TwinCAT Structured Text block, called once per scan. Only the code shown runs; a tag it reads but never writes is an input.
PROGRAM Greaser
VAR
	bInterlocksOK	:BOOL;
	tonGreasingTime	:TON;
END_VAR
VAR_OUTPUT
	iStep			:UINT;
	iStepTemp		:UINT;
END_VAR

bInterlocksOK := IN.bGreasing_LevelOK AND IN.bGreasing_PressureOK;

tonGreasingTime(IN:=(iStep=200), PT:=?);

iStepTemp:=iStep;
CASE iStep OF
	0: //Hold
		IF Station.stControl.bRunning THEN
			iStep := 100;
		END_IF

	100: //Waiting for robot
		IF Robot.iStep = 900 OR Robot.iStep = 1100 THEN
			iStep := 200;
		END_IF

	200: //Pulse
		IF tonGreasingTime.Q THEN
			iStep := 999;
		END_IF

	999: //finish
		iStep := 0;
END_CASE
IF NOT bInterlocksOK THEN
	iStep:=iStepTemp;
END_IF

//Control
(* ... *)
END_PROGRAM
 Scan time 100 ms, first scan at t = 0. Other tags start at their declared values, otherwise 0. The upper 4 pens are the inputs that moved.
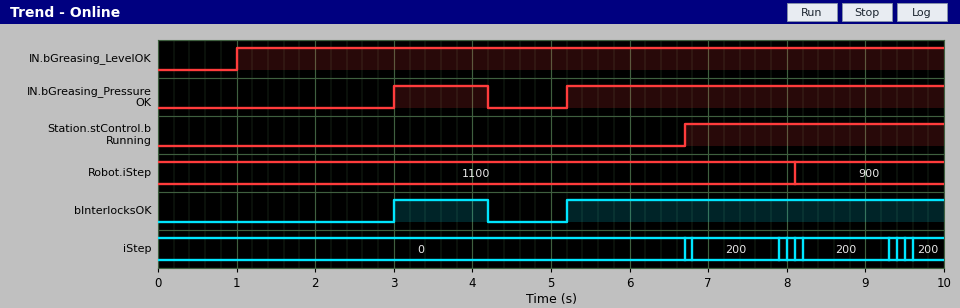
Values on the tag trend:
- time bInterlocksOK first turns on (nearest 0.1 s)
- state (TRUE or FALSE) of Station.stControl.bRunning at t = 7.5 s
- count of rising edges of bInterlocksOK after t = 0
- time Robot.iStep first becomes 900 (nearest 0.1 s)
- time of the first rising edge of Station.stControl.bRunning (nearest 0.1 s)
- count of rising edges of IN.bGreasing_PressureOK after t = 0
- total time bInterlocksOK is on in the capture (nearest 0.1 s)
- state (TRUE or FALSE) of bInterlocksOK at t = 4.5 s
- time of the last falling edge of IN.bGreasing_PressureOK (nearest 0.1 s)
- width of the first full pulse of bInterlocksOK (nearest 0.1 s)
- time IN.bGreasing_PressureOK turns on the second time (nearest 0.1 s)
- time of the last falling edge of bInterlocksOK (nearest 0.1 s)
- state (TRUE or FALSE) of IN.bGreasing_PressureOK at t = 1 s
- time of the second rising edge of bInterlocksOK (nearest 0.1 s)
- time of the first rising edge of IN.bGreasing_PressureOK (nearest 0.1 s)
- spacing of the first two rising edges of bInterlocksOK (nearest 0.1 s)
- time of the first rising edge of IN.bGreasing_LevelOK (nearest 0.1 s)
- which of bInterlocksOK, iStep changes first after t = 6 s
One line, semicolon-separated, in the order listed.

3.0 s; TRUE; 2; 8.1 s; 6.7 s; 2; 6.0 s; FALSE; 4.2 s; 1.2 s; 5.2 s; 4.2 s; FALSE; 5.2 s; 3.0 s; 2.2 s; 1.0 s; iStep
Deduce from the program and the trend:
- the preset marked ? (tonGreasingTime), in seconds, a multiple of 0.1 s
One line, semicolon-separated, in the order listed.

1.0 s
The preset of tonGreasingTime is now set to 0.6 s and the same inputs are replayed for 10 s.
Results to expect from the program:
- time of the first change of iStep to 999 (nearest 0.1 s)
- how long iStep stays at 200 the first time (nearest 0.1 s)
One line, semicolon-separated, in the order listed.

7.5 s; 0.7 s
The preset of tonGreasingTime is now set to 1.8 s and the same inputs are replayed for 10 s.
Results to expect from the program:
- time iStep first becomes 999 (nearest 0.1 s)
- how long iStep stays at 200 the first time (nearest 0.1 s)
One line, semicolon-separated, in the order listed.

8.7 s; 1.9 s
